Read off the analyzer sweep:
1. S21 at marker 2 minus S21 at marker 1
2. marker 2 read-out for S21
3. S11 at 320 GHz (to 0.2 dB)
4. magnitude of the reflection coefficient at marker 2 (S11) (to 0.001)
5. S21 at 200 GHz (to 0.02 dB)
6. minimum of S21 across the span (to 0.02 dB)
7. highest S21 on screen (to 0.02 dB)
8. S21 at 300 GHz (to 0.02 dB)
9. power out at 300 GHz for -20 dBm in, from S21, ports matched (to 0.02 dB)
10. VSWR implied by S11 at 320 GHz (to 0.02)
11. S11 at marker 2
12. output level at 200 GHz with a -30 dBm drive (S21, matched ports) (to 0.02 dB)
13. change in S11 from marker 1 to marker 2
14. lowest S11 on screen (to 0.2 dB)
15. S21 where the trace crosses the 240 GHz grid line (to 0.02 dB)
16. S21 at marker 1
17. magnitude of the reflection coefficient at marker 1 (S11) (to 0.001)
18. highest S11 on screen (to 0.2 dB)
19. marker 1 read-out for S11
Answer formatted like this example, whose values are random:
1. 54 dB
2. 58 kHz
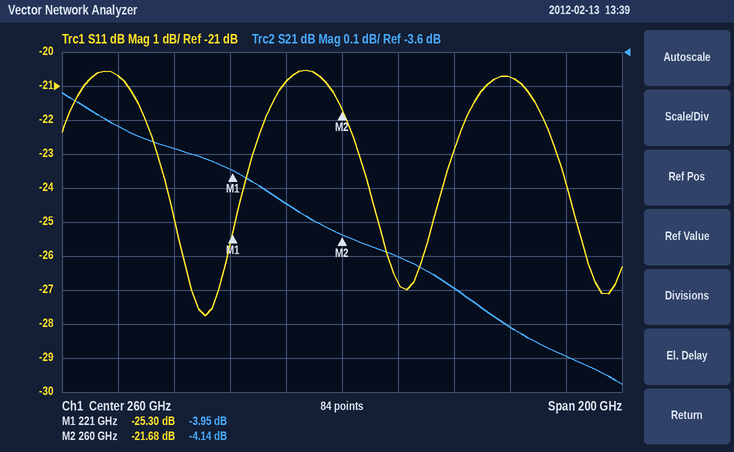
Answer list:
1. -0.19 dB
2. -4.14 dB
3. -20.8 dB
4. 0.082
5. -3.88 dB
6. -4.58 dB
7. -3.72 dB
8. -4.30 dB
9. -24.30 dBm
10. 1.20
11. -21.68 dB
12. -33.88 dBm
13. 3.62 dB
14. -27.8 dB
15. -4.04 dB
16. -3.95 dB
17. 0.054
18. -20.6 dB
19. -25.30 dB
